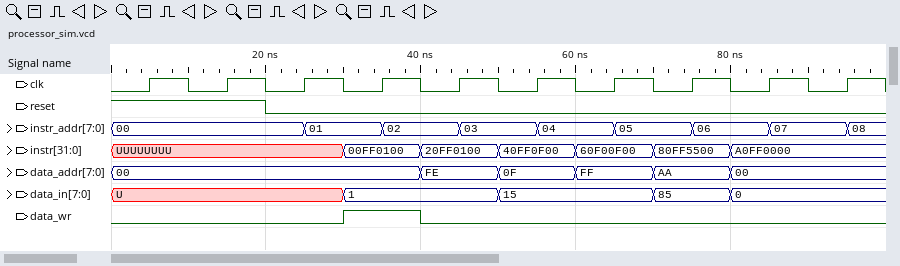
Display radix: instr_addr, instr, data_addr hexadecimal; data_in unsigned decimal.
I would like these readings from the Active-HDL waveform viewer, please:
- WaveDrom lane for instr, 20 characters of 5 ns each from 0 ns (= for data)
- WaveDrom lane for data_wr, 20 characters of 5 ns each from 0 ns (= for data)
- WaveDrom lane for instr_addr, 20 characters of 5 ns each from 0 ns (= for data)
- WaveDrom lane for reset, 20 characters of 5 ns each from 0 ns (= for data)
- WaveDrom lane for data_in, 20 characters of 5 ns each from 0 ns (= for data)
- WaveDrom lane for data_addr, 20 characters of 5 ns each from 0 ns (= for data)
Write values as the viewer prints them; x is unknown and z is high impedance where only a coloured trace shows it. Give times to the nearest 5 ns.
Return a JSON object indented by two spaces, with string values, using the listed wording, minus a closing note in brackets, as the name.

{
  "WaveDrom lane for instr, 20 characters of 5 ns each from 0 ns": "{name: 'instr', wave: 'x.....=.=.=.=.=.=...', data: '00FF0100 20FF0100 40FF0F00 60F00F00 80FF5500 A0FF0000'}",
  "WaveDrom lane for data_wr, 20 characters of 5 ns each from 0 ns": "{name: 'data_wr', wave: '0.....1.0...........'}",
  "WaveDrom lane for instr_addr, 20 characters of 5 ns each from 0 ns": "{name: 'instr_addr', wave: '=....=.=.=.=.=.=.=.=', data: '00 01 02 03 04 05 06 07 08'}",
  "WaveDrom lane for reset, 20 characters of 5 ns each from 0 ns": "{name: 'reset', wave: '1...0...............'}",
  "WaveDrom lane for data_in, 20 characters of 5 ns each from 0 ns": "{name: 'data_in', wave: 'x.....=...=...=.=...', data: '1 15 85 0'}",
  "WaveDrom lane for data_addr, 20 characters of 5 ns each from 0 ns": "{name: 'data_addr', wave: '=.......=.=.=.=.=...', data: '00 FE 0F FF AA 00'}"
}
